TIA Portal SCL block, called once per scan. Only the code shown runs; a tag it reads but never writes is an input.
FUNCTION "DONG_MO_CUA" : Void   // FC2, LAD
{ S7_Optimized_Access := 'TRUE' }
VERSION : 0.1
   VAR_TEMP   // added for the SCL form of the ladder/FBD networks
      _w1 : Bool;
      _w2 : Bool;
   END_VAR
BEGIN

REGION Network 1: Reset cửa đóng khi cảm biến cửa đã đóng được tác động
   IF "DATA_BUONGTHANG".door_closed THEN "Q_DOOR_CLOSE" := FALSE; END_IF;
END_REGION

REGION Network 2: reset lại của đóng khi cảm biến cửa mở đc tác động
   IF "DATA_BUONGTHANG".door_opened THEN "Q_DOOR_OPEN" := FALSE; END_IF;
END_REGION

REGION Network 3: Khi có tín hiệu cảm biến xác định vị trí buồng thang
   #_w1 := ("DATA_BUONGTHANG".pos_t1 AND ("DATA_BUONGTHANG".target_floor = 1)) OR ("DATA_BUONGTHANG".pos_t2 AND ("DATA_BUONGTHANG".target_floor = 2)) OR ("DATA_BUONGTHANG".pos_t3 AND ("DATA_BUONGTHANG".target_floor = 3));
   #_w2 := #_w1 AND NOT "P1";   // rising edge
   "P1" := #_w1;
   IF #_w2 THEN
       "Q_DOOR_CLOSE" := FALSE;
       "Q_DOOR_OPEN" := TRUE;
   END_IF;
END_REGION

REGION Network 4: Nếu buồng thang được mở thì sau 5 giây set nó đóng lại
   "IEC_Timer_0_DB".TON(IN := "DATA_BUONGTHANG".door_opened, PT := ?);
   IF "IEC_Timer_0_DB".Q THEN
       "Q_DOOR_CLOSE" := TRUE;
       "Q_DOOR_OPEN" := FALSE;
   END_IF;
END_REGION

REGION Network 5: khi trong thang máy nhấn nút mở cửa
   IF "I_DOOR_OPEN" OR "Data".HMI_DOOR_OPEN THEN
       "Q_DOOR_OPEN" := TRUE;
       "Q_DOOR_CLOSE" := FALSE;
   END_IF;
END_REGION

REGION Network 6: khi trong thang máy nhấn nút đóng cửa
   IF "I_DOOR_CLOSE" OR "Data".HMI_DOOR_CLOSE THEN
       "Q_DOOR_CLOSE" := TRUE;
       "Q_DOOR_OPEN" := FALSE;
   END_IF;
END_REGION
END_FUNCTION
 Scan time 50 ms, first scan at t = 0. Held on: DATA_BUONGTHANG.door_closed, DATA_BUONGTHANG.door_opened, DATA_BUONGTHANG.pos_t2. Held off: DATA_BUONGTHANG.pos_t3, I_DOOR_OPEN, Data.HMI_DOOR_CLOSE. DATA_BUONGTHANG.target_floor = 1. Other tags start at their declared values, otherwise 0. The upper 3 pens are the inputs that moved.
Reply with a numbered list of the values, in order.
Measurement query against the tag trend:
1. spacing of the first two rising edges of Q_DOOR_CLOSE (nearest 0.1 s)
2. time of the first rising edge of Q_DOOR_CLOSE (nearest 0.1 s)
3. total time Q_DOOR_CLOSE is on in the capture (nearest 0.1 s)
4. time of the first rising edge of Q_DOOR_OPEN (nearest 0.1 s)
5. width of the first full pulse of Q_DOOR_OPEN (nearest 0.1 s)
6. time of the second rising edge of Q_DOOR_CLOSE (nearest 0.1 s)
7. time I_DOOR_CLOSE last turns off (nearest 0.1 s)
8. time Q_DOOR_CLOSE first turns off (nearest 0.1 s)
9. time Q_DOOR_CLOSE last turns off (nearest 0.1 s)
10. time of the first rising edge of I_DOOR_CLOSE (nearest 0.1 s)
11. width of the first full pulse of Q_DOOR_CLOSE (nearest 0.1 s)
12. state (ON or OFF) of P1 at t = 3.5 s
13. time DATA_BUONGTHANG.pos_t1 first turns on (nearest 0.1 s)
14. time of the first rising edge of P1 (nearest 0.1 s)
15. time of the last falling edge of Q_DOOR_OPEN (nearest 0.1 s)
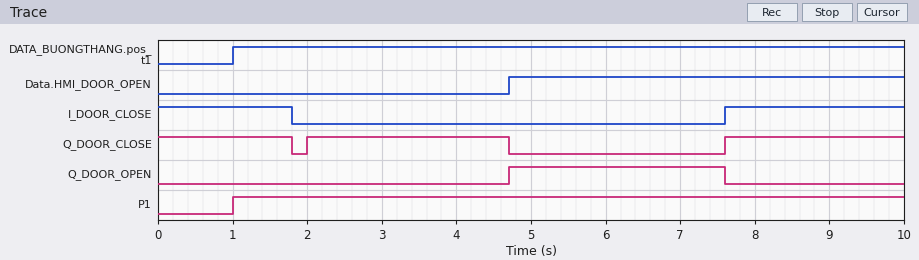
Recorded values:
1. 5.6 s
2. 2.0 s
3. 6.9 s
4. 4.7 s
5. 2.9 s
6. 7.6 s
7. 1.8 s
8. 1.8 s
9. 4.7 s
10. 7.6 s
11. 2.7 s
12. ON
13. 1.0 s
14. 1.0 s
15. 7.6 s
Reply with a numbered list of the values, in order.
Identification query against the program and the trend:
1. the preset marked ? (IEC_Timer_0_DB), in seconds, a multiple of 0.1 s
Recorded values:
1. 2.0 s
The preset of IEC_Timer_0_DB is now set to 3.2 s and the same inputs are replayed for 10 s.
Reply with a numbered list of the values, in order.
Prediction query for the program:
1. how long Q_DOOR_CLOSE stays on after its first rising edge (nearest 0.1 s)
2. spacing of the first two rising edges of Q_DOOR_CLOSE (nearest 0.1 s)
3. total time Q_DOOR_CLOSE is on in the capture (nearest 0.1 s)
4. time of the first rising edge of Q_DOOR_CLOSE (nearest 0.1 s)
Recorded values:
1. 1.5 s
2. 4.4 s
3. 5.7 s
4. 3.2 s
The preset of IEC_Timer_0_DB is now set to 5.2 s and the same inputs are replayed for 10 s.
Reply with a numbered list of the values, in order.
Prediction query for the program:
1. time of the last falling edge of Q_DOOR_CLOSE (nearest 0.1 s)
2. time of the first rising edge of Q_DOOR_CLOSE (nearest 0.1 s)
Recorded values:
1. 1.8 s
2. 7.6 s
